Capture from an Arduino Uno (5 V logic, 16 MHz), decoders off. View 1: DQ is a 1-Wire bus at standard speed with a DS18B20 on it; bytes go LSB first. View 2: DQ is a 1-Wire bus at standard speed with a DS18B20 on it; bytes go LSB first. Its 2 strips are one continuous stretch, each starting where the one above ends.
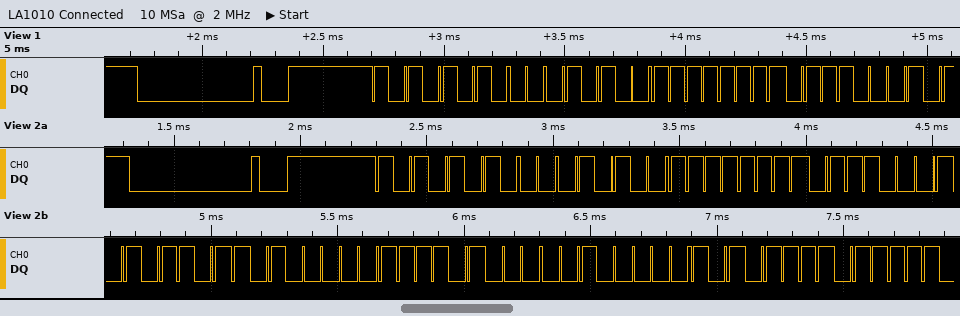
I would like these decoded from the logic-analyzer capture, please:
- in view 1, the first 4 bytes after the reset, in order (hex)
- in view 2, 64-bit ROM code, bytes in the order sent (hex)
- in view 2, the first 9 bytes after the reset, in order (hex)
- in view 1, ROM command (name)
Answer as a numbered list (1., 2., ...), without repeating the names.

1. 55 28 FF 8E
2. 28 FF 8E DA 82 17 04 F5
3. 55 28 FF 8E DA 82 17 04 F5
4. Match ROM
